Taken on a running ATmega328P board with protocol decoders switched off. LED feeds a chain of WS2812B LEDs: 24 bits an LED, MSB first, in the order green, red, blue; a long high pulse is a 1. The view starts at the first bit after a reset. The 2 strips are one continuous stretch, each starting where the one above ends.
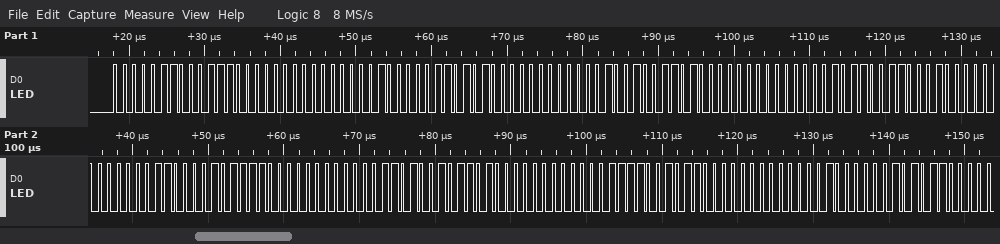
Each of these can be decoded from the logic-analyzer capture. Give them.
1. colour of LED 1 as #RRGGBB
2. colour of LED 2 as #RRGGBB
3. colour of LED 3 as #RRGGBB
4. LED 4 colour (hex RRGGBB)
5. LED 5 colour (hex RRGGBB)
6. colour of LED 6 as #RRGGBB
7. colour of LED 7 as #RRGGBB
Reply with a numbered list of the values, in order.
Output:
1. #380600
2. #350800
3. #340900
4. #310B00
5. #2F0C00
6. #2D0D00
7. #2C0F00
